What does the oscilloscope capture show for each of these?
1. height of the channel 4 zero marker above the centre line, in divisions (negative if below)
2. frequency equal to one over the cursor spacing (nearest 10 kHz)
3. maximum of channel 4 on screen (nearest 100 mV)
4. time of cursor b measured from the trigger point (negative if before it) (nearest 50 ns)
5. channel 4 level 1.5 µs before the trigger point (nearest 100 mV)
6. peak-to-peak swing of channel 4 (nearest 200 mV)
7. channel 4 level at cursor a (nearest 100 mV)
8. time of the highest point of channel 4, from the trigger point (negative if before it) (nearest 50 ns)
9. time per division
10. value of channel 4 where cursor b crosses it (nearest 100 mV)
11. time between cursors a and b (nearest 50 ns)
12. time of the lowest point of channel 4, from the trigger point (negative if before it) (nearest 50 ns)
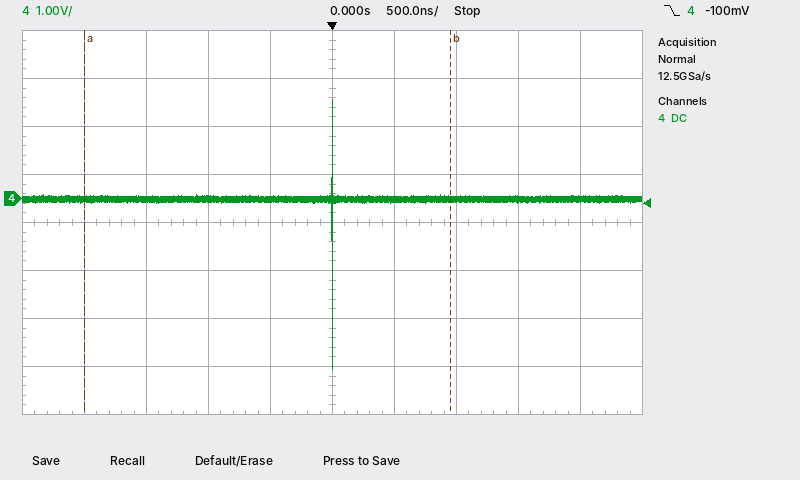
+0.5 div
340 kHz
2.1 V
+950 ns
0.0 V
5.6 V
0.0 V
0 ns
500 ns
0.0 V
2.95 µs
0 ns
